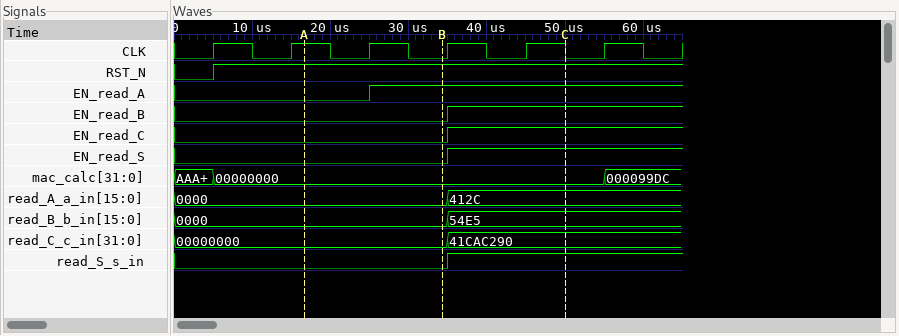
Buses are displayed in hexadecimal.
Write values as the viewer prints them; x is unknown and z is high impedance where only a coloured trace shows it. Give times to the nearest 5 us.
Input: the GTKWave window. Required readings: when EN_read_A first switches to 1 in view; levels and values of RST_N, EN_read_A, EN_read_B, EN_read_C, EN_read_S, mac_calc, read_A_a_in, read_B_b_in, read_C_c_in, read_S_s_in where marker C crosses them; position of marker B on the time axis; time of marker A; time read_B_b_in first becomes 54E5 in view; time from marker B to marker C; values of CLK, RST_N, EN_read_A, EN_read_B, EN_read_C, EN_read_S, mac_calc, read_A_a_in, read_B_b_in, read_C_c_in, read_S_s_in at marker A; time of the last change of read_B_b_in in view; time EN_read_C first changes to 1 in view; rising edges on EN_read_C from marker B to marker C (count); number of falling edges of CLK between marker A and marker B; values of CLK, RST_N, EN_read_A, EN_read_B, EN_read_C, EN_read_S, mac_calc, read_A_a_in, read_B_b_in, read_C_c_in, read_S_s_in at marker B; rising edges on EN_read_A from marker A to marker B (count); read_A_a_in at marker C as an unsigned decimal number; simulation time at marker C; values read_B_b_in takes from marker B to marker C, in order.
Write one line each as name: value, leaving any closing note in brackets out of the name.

when EN_read_A first switches to 1 in view: 25 us
levels and values of RST_N, EN_read_A, EN_read_B, EN_read_C, EN_read_S, mac_calc, read_A_a_in, read_B_b_in, read_C_c_in, read_S_s_in where marker C crosses them: RST_N=1, EN_read_A=1, EN_read_B=1, EN_read_C=1, EN_read_S=1, mac_calc=00000000, read_A_a_in=412C, read_B_b_in=54E5, read_C_c_in=41CAC290, read_S_s_in=1
position of marker B on the time axis: 35 us
time of marker A: 15 us
time read_B_b_in first becomes 54E5 in view: 35 us
time from marker B to marker C: 15 us
values of CLK, RST_N, EN_read_A, EN_read_B, EN_read_C, EN_read_S, mac_calc, read_A_a_in, read_B_b_in, read_C_c_in, read_S_s_in at marker A: CLK=1, RST_N=1, EN_read_A=0, EN_read_B=0, EN_read_C=0, EN_read_S=0, mac_calc=00000000, read_A_a_in=0000, read_B_b_in=0000, read_C_c_in=00000000, read_S_s_in=0
time of the last change of read_B_b_in in view: 35 us
time EN_read_C first changes to 1 in view: 35 us
rising edges on EN_read_C from marker B to marker C: 1
number of falling edges of CLK between marker A and marker B: 2
values of CLK, RST_N, EN_read_A, EN_read_B, EN_read_C, EN_read_S, mac_calc, read_A_a_in, read_B_b_in, read_C_c_in, read_S_s_in at marker B: CLK=0, RST_N=1, EN_read_A=1, EN_read_B=0, EN_read_C=0, EN_read_S=0, mac_calc=00000000, read_A_a_in=0000, read_B_b_in=0000, read_C_c_in=00000000, read_S_s_in=0
rising edges on EN_read_A from marker A to marker B: 1
read_A_a_in at marker C as an unsigned decimal number: 16684
simulation time at marker C: 50 us
values read_B_b_in takes from marker B to marker C, in order: 0000, 54E5
